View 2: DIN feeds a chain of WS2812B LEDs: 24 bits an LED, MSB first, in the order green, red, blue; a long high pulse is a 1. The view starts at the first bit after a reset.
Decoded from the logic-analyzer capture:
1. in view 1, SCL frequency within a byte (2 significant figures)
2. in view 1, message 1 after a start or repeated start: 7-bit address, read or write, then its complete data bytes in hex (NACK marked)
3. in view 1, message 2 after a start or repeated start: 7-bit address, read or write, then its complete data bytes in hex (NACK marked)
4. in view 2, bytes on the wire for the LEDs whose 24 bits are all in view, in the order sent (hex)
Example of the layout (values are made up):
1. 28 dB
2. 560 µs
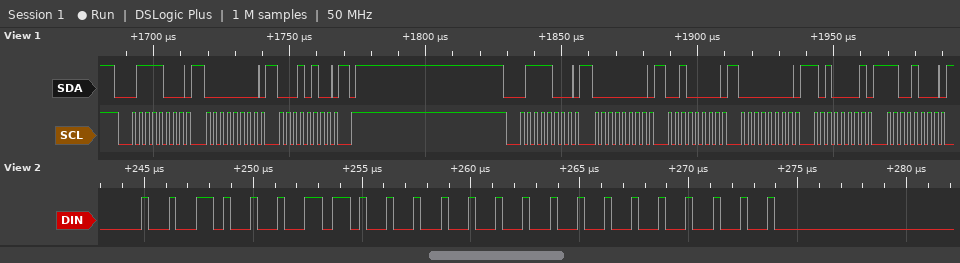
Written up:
1. 400 kHz
2. 0x3C write: 00 14
3. 0x3C write: 00 20 00 A1 C8
4. 23 00 00
